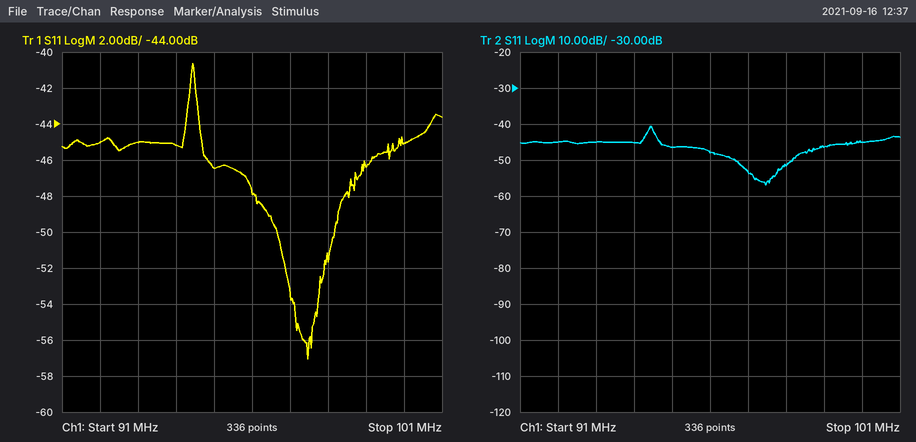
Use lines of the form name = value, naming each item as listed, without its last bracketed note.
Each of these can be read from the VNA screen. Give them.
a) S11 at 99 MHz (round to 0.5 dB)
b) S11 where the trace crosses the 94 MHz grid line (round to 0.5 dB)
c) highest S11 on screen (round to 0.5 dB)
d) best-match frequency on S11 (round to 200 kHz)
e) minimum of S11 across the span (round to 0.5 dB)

S11 at 99 MHz = -46.5 dB
S11 where the trace crosses the 94 MHz grid line = -45.0 dB
highest S11 on screen = -40.5 dB
best-match frequency on S11 = 97.4 MHz
minimum of S11 across the span = -57.0 dB
